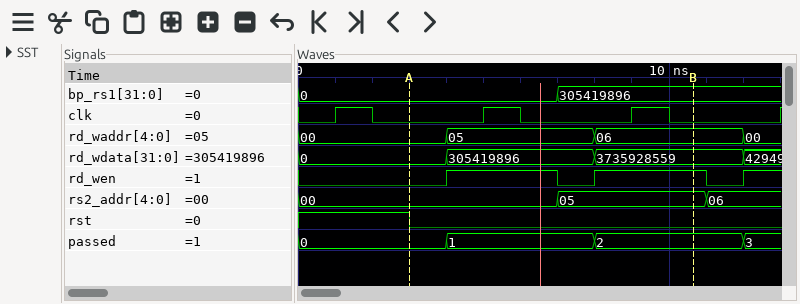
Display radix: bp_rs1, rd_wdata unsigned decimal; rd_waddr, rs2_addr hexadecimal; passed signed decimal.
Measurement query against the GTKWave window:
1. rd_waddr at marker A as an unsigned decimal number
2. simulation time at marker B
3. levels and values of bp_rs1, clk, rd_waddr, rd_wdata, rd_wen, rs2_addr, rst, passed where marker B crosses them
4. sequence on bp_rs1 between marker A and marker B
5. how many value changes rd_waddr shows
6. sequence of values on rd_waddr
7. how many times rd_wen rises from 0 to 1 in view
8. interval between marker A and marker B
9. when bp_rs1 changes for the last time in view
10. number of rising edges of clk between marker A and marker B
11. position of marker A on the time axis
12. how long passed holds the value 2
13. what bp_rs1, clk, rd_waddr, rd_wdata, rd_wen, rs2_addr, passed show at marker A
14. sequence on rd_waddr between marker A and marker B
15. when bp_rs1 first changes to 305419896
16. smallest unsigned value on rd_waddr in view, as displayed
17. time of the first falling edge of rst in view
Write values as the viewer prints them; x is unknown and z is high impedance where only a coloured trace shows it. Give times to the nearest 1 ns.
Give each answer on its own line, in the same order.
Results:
0
11 ns
bp_rs1=305419896, clk=0, rd_waddr=06, rd_wdata=3735928559, rd_wen=1, rs2_addr=05, rst=0, passed=2
0, 305419896
3
00, 05, 06, 00
3
8 ns
7 ns
2
3 ns
4 ns
bp_rs1=0, clk=0, rd_waddr=00, rd_wdata=0, rd_wen=0, rs2_addr=00, passed=0
00, 05, 06
7 ns
00
3 ns
